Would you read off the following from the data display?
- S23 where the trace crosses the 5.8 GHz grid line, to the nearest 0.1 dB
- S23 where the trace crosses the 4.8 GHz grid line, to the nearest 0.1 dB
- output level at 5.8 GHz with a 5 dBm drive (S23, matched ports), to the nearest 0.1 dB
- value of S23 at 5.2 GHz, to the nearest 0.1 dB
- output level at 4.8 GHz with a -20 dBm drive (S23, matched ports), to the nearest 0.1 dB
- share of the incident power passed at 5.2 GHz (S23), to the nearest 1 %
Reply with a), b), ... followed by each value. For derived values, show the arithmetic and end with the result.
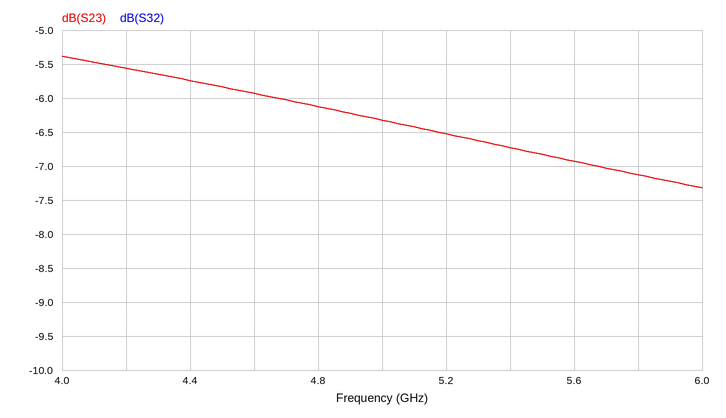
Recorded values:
a) -7.1 dB
b) -6.1 dB
c) 5 dBm + (-7.1 dB) = -2.1 dBm
d) -6.5 dB
e) -20 dBm + (-6.1 dB) = -26.1 dBm
f) 10^(-6.5/10) ≈ 22 %
